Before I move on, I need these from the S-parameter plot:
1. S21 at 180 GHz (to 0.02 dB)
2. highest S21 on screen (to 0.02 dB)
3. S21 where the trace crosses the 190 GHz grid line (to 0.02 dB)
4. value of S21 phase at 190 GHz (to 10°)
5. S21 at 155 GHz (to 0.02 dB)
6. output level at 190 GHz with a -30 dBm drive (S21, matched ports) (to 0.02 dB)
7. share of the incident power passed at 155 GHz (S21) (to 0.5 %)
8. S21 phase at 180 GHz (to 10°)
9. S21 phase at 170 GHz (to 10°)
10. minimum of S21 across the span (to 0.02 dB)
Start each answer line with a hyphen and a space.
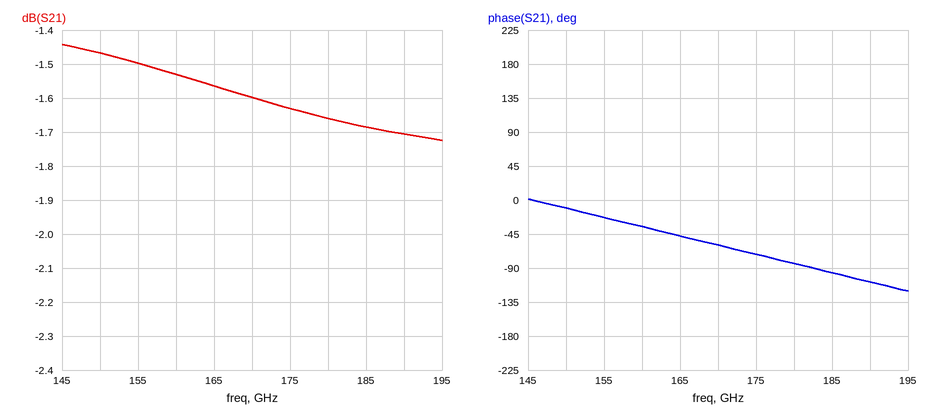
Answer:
- -1.66 dB
- -1.44 dB
- -1.70 dB
- -110°
- -1.50 dB
- -31.70 dBm
- 71.0 %
- -80°
- -60°
- -1.72 dB
